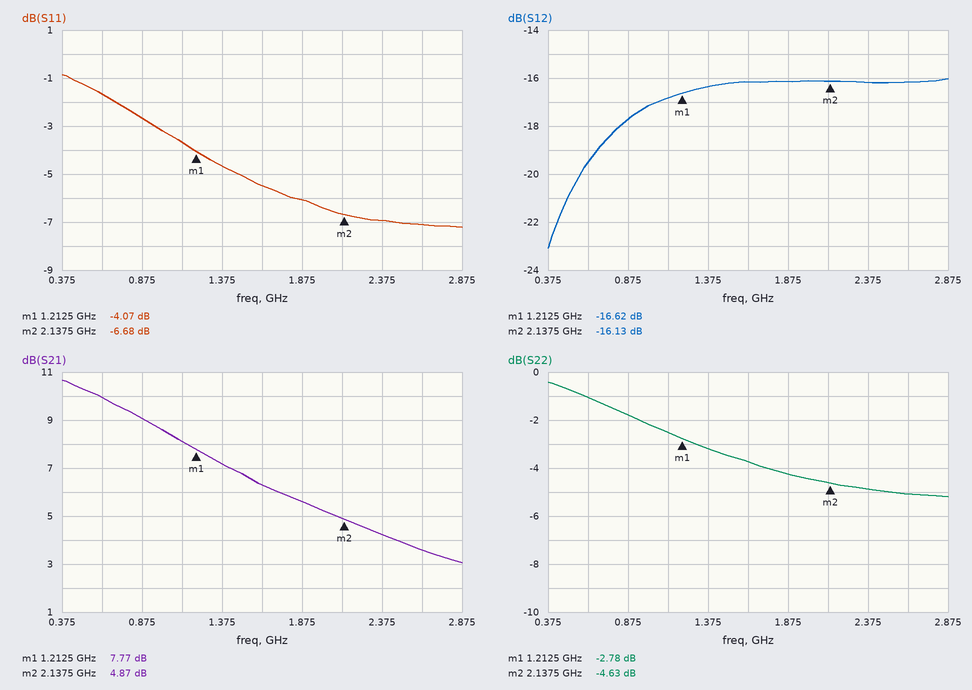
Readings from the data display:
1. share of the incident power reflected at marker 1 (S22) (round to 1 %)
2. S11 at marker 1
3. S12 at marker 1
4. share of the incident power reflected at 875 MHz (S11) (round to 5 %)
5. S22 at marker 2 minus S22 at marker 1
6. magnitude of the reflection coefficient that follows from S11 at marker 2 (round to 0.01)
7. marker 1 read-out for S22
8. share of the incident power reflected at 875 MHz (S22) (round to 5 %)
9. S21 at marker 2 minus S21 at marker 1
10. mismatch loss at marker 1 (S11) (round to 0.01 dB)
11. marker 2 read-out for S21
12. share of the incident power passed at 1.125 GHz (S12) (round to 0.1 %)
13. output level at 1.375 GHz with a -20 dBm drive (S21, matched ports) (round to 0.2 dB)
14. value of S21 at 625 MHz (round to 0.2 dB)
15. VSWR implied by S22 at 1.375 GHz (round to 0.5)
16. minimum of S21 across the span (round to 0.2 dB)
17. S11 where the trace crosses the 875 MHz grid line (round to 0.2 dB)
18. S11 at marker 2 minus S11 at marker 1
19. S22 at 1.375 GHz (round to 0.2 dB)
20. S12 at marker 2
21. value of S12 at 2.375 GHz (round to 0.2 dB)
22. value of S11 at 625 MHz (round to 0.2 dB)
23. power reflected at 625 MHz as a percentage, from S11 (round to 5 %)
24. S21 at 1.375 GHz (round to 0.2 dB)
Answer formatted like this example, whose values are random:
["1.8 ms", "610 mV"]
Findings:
["53 %", "-4.07 dB", "-16.62 dB", "55 %", "-1.85 dB", "0.46", "-2.78 dB", "65 %", "-2.90 dB", "2.16 dB", "4.87 dB", "2.1 %", "-12.8 dBm", "10.0 dB", "5.5", "3.0 dB", "-2.6 dB", "-2.61 dB", "-3.2 dB", "-16.13 dB", "-16.2 dB", "-1.6 dB", "70 %", "7.2 dB"]
